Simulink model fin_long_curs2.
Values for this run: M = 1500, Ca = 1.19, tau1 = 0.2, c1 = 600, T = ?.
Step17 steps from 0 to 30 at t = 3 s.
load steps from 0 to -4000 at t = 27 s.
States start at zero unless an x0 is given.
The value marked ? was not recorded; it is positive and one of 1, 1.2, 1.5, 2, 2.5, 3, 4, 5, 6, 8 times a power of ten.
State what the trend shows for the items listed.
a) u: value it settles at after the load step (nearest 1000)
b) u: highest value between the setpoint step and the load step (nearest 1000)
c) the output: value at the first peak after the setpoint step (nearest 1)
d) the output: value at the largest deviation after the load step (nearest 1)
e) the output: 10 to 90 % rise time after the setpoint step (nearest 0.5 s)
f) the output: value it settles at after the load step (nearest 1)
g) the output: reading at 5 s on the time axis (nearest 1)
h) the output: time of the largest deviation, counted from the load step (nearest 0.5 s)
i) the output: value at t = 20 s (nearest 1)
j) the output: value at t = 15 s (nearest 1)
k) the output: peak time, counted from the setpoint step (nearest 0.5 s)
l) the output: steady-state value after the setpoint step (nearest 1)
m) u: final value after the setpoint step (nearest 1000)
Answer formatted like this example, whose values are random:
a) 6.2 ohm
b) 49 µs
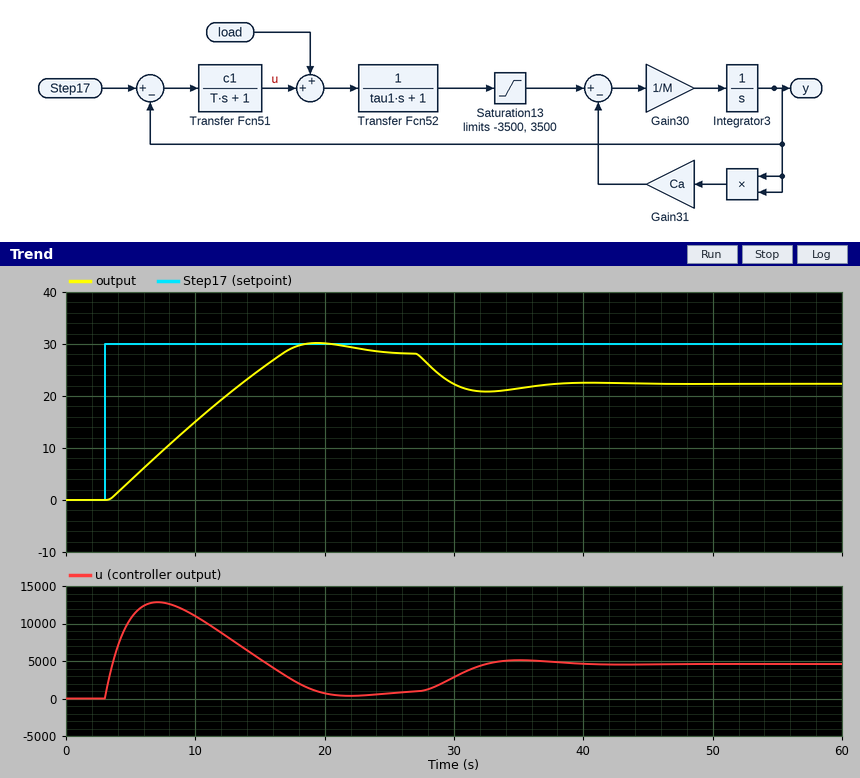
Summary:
a) 5000
b) 13000
c) 30
d) 21
e) 10.5 s
f) 22
g) 4
h) 5.5 s
i) 30
j) 25
k) 16.5 s
l) 28
m) 1000
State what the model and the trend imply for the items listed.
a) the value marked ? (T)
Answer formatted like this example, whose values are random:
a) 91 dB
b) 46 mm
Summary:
a) 2
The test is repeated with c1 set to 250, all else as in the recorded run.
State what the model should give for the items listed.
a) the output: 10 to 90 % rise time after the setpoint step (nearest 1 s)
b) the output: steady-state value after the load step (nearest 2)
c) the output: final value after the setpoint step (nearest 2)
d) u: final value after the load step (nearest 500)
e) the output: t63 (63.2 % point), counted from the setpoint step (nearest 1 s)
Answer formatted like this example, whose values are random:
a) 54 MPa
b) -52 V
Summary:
a) 10 s
b) 14
c) 26
d) 4000
e) 8 s
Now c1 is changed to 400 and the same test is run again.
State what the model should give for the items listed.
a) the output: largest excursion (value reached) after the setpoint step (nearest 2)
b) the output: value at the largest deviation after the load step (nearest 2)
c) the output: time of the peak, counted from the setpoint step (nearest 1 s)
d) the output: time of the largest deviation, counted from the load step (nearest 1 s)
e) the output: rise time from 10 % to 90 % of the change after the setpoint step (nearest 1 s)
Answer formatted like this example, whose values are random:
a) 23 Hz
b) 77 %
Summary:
a) 28
b) 18
c) 17 s
d) 8 s
e) 10 s
